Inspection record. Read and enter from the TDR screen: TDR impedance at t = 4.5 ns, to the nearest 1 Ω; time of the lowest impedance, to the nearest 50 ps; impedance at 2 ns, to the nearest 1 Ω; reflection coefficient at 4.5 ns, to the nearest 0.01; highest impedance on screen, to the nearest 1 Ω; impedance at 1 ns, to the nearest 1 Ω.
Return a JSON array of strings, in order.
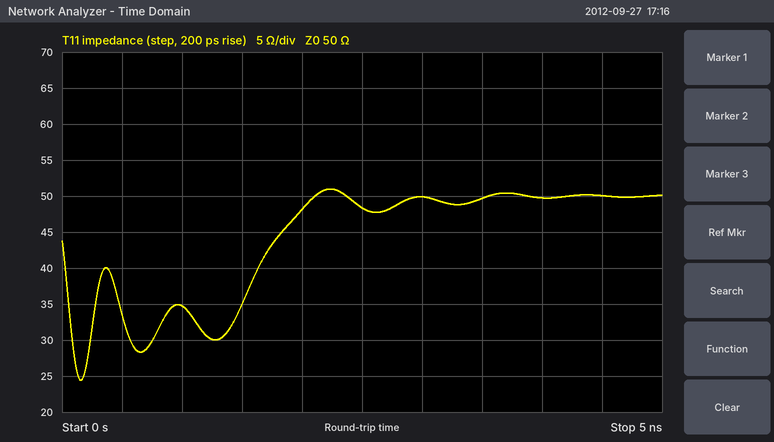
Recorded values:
["50 Ω", "150 ps", "48 Ω", "0.00", "51 Ω", "35 Ω"]
